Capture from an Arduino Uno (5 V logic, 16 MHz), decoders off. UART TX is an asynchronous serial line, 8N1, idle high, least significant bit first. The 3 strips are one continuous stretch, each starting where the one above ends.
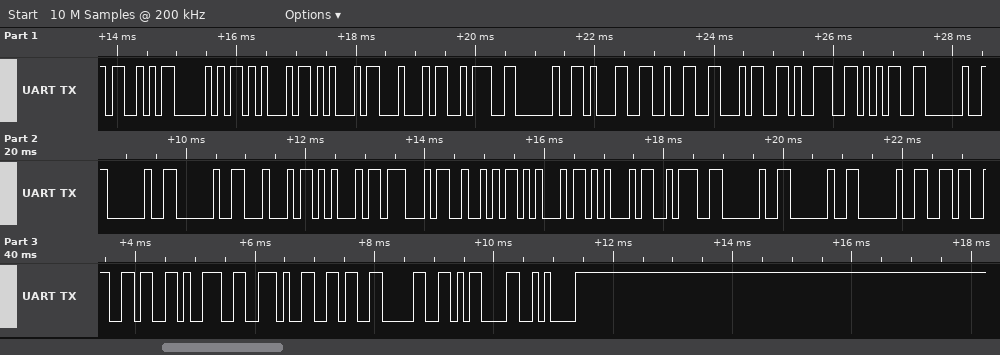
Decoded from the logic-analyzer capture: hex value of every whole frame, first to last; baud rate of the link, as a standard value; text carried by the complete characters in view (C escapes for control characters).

53 50 45 45 44 3A 20 31 32 34 39 35 20 20 20 44 45 47 52 45 45 3A 20 20 20 36 36 39 2E 36 30 0D 0A
9600 baud
"SPEED: 12495   DEGREE:   669.60\r\n"
